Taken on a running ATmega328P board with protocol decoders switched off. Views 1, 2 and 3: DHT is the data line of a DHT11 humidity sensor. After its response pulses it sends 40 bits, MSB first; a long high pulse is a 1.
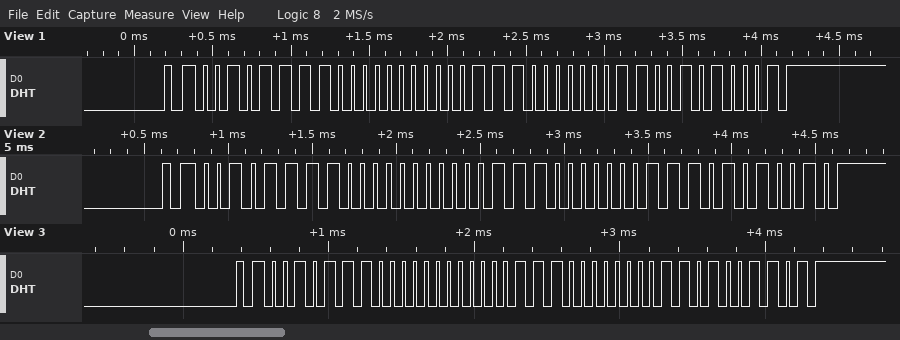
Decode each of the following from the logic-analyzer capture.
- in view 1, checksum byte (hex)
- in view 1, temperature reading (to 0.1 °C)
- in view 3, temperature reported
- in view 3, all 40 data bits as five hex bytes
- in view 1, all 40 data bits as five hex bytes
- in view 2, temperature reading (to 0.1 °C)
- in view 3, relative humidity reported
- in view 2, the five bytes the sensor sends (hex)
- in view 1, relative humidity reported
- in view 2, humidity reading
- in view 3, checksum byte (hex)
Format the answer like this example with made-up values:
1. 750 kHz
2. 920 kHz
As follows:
1. 0x51
2. 28.6 °C
3. 28.3 °C
4. 2E 00 1C 03 4D
5. 2F 00 1C 06 51
6. 28.7 °C
7. 46 %
8. 2F 00 1C 07 52
9. 47 %
10. 47 %
11. 0x4D
